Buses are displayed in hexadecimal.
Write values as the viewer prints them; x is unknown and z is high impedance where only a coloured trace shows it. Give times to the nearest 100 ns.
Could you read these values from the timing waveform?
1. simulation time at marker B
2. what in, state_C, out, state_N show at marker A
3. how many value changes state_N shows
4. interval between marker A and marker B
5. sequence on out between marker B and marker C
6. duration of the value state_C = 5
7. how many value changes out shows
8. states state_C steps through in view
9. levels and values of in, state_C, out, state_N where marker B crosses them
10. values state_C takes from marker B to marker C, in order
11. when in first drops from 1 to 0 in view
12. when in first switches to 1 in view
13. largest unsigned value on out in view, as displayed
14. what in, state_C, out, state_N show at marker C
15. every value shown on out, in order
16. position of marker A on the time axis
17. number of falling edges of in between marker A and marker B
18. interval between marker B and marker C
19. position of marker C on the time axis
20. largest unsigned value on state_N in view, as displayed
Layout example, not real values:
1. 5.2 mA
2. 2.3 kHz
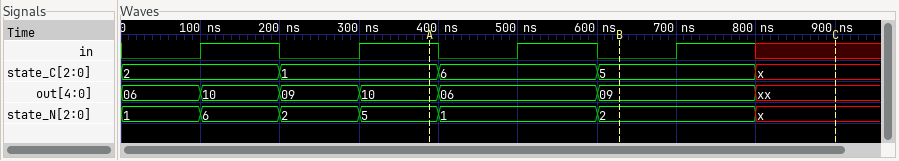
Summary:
1. 600 ns
2. in=1, state_C=1, out=10, state_N=5
3. 6
4. 200 ns
5. 09, xx
6. 200 ns
7. 6
8. 2, 1, 6, 5, x
9. in=0, state_C=5, out=09, state_N=2
10. 5, x
11. 200 ns
12. 100 ns
13. 10
14. in=x, state_C=x, out=xx, state_N=x
15. 06, 10, 09, 10, 06, 09, xx
16. 400 ns
17. 2
18. 300 ns
19. 900 ns
20. 6
